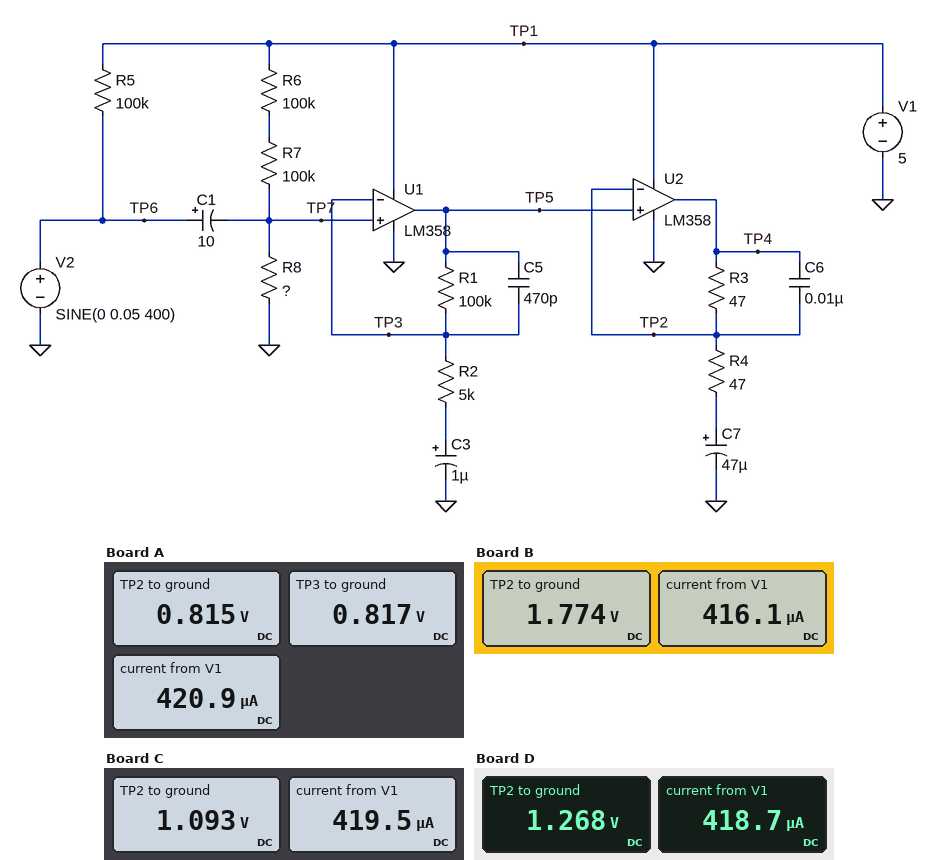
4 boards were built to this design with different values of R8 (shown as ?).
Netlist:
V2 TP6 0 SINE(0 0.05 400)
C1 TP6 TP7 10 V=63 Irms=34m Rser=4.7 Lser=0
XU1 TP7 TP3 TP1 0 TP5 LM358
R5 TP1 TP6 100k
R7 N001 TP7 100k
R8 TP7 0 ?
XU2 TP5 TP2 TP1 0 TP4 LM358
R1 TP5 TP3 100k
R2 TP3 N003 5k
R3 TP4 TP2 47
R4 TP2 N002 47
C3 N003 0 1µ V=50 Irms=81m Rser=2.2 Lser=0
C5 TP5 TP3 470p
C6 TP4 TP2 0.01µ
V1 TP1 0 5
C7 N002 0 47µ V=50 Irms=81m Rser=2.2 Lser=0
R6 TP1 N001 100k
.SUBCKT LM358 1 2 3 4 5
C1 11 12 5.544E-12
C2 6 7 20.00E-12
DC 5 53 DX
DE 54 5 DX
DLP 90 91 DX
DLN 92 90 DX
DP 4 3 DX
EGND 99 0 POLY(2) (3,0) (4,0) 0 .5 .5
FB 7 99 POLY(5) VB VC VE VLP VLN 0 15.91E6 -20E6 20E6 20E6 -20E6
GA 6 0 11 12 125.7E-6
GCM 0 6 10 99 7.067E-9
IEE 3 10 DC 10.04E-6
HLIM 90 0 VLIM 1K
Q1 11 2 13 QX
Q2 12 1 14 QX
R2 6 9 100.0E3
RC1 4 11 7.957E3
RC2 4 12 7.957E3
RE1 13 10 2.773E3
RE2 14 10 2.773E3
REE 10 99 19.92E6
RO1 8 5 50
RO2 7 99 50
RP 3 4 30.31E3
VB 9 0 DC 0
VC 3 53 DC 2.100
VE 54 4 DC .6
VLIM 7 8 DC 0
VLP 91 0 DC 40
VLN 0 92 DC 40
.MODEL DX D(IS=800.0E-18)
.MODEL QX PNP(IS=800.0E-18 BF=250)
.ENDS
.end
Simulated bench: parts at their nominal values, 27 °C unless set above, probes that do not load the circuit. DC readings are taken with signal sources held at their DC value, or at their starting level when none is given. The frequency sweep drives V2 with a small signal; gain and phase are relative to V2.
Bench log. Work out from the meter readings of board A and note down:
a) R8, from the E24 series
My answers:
39 kΩ
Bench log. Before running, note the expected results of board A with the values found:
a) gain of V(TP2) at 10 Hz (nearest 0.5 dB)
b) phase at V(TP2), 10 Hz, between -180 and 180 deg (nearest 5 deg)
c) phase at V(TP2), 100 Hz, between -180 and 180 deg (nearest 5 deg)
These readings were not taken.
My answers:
16.0 dB
65 deg
15 deg
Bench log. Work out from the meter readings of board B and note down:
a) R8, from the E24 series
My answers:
110 kΩ
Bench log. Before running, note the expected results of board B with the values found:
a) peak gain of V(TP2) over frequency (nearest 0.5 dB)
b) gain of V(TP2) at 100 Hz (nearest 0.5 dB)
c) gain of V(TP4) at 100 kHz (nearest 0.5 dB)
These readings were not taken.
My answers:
26.5 dB
26.0 dB
6.5 dB
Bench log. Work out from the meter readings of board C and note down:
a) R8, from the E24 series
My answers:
56 kΩ
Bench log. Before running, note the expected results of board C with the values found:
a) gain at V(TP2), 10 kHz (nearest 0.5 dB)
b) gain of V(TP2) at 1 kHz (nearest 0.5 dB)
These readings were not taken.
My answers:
16.0 dB
26.0 dB
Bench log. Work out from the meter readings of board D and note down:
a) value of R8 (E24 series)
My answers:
68 kΩ
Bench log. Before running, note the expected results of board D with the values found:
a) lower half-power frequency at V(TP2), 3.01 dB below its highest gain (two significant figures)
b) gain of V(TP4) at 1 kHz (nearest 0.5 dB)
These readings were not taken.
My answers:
31 Hz
32.0 dB
